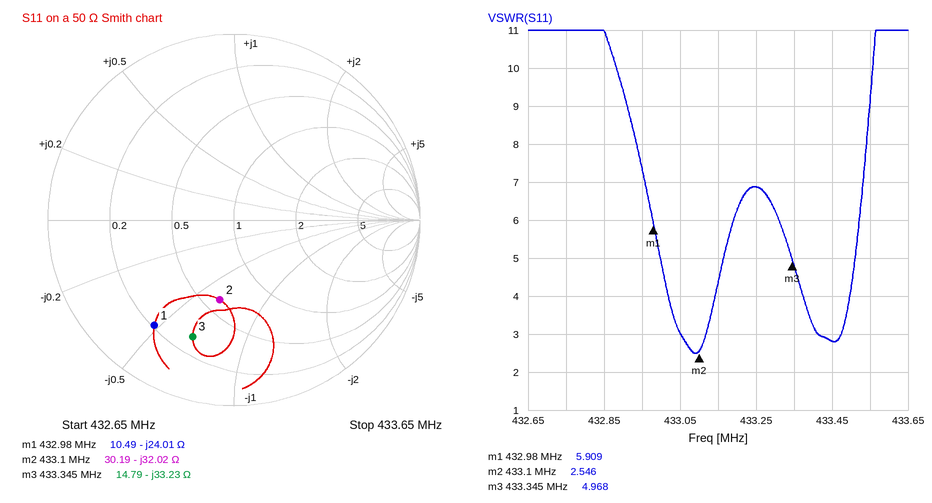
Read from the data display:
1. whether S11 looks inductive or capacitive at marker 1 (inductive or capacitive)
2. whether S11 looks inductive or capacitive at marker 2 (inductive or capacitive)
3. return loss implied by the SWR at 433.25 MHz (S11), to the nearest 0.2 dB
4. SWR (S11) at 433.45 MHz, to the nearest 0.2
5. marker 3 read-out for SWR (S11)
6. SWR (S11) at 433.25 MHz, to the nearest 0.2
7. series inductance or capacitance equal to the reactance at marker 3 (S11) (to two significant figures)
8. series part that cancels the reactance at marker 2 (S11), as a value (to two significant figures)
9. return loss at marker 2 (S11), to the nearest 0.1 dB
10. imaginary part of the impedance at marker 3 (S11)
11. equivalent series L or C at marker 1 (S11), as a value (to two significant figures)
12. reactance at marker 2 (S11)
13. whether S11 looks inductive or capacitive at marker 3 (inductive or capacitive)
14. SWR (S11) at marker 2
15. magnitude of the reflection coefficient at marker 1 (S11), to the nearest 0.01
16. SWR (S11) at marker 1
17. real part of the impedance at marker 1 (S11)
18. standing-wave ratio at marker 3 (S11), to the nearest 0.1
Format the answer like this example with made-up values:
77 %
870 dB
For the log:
capacitive
capacitive
2.6 dB
2.8
4.968
6.8
11 pF
12 nH
7.2 dB
-33.23 Ω
15 pF
-32.02 Ω
capacitive
2.546
0.71
5.909
10.49 Ω
5.0
